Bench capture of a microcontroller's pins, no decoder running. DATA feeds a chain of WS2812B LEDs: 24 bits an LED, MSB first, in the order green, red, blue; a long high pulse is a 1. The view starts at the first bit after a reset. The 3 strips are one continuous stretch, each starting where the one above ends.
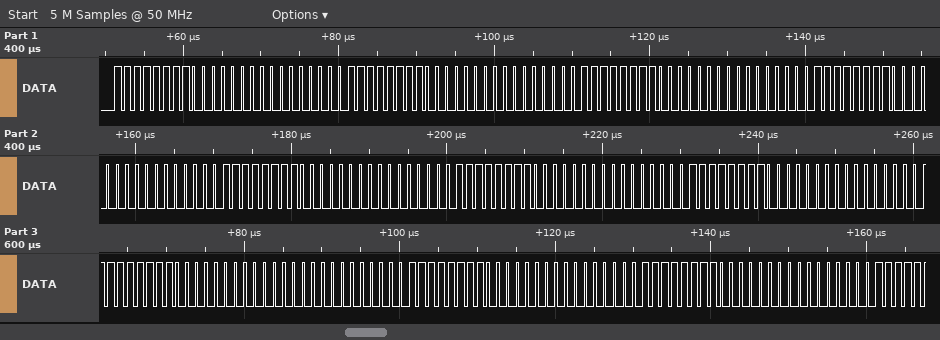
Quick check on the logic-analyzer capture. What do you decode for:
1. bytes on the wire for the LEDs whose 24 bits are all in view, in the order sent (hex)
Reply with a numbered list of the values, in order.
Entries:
1. FF 00 00 FF 00 00 FF 00 00 FF 00 00 FF 00 00 FF 00 00 FF 00 00 FF 00 00 00 FF 00 00 FF 00
